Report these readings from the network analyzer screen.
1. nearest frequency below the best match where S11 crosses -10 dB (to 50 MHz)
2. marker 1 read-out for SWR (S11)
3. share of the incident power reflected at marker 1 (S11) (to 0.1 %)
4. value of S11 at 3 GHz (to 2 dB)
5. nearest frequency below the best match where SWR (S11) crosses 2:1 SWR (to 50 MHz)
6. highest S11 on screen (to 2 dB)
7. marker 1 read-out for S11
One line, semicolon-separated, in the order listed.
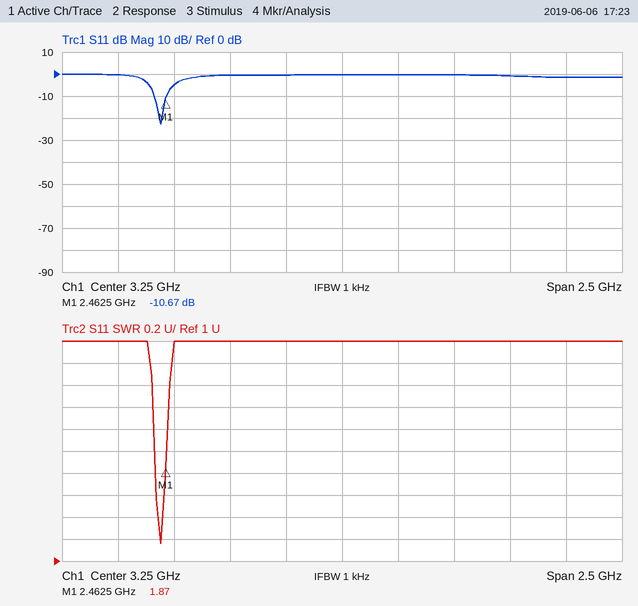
2.40 GHz; 1.87; 8.6 %; 0 dB; 2.40 GHz; 0 dB; -10.67 dB
